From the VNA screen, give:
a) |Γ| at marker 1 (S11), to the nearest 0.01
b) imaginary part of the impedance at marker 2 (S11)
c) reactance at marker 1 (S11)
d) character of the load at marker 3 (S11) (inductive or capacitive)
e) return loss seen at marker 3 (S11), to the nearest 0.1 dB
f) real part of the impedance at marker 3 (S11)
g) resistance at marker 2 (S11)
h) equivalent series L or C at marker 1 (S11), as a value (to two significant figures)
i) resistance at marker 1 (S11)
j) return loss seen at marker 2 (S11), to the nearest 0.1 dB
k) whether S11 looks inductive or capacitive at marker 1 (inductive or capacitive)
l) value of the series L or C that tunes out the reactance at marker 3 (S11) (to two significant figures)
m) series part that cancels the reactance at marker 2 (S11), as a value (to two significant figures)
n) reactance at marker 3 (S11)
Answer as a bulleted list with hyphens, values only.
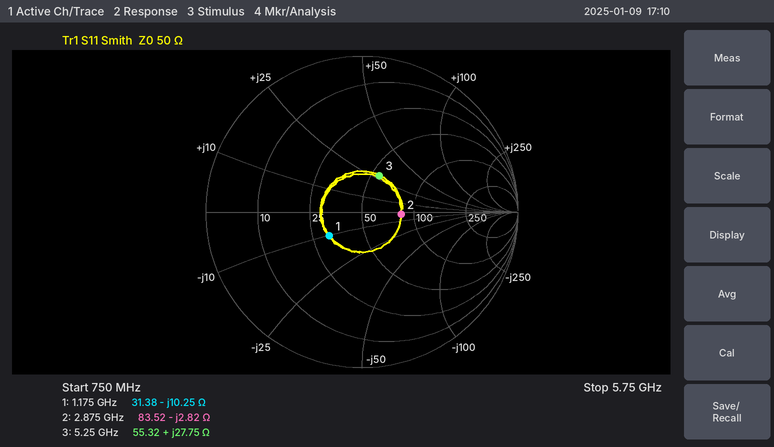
- 0.26
- -2.82 Ω
- -10.25 Ω
- inductive
- 11.7 dB
- 55.32 Ω
- 83.52 Ω
- 13 pF
- 31.38 Ω
- 12.0 dB
- capacitive
- 1.1 pF
- 160 pH
- +27.75 Ω
